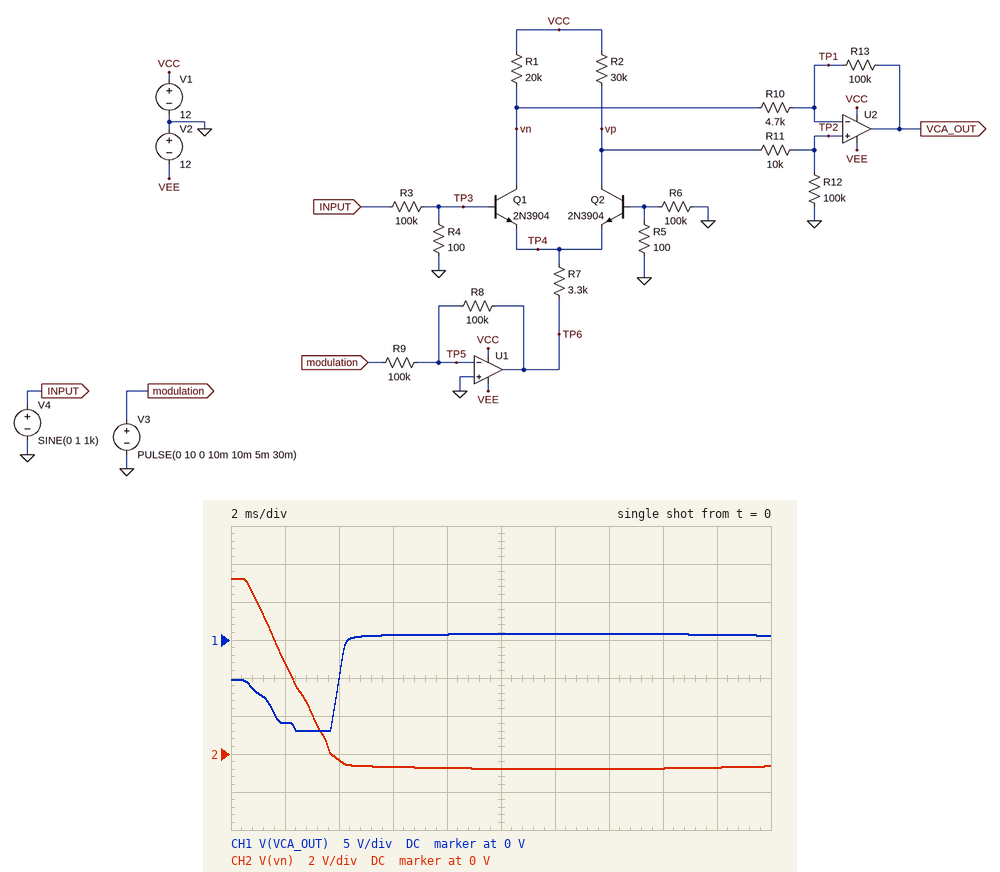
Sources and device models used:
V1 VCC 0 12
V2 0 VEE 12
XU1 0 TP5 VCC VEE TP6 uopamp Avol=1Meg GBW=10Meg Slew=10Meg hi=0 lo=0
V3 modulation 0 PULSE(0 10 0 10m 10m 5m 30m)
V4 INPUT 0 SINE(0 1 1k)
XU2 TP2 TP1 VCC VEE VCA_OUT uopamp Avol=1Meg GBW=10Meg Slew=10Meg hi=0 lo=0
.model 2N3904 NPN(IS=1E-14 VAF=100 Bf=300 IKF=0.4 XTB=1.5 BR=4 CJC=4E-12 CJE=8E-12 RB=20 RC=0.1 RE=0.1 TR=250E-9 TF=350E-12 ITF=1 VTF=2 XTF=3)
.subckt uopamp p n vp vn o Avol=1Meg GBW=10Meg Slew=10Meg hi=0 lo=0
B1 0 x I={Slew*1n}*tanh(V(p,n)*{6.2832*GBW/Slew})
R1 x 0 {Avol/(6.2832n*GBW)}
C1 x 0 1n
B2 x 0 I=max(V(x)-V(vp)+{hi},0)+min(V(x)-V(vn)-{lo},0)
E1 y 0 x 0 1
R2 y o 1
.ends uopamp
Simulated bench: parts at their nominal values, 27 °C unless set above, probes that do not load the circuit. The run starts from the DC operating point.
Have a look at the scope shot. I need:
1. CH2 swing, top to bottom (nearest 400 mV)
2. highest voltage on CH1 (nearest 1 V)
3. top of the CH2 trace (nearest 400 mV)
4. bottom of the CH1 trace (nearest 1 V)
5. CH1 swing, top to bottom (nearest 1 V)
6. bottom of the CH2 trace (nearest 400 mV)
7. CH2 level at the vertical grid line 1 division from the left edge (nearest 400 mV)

10.0 V
1 V
9.2 V
-12 V
13 V
-800 mV
4.8 V
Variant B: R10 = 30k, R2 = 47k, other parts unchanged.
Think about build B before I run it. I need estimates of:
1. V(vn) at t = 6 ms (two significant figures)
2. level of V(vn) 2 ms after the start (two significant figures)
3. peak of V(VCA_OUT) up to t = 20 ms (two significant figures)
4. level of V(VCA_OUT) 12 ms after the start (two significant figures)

-700 mV
5.2 V
-440 mV
-490 mV
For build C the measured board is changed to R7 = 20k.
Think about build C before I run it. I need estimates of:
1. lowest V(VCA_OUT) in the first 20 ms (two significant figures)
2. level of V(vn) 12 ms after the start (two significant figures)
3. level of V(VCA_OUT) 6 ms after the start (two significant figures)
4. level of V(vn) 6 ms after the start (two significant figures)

-12 V
4.3 V
-9.0 V
6.4 V
